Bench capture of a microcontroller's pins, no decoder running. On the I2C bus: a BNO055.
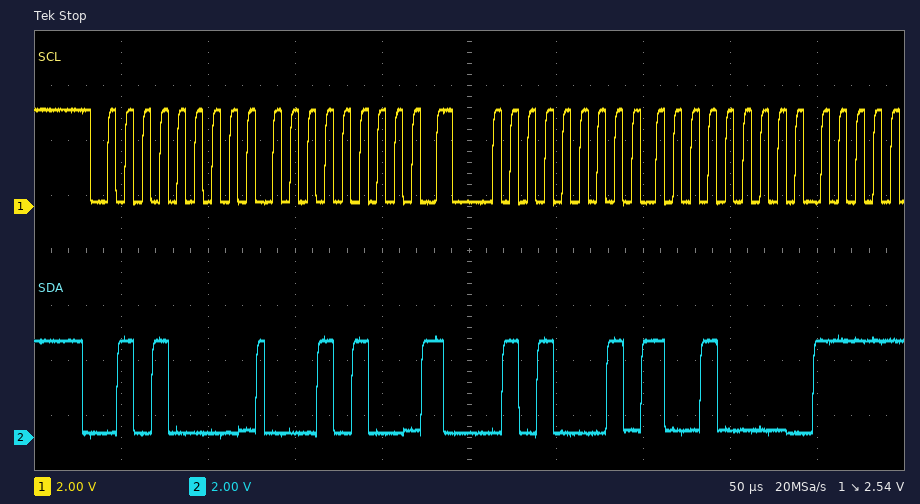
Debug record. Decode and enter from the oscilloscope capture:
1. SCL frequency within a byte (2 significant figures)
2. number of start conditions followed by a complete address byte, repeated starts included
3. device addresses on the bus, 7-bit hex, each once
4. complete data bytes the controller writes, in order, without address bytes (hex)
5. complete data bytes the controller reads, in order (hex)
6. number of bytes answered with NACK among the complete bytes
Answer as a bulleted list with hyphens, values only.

- 100 kHz
- 2
- 0x28
- 14
- 90
- 0
